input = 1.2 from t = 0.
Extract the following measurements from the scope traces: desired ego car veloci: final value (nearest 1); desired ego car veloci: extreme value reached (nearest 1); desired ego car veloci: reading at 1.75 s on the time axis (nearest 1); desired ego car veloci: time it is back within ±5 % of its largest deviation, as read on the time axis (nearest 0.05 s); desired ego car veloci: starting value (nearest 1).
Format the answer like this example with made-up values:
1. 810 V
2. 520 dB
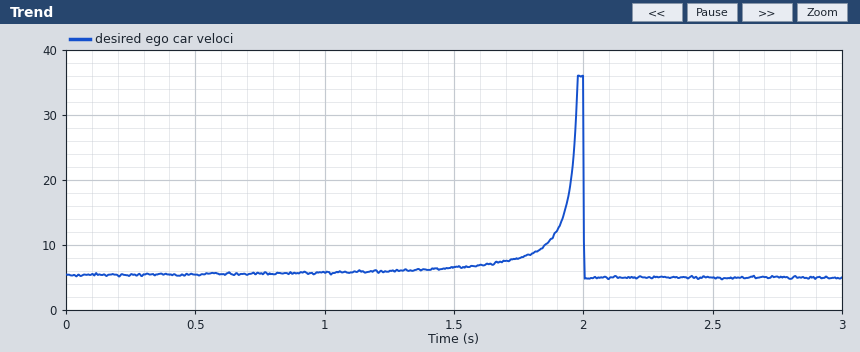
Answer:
1. 5
2. 36
3. 8
4. 2.00 s
5. 5
